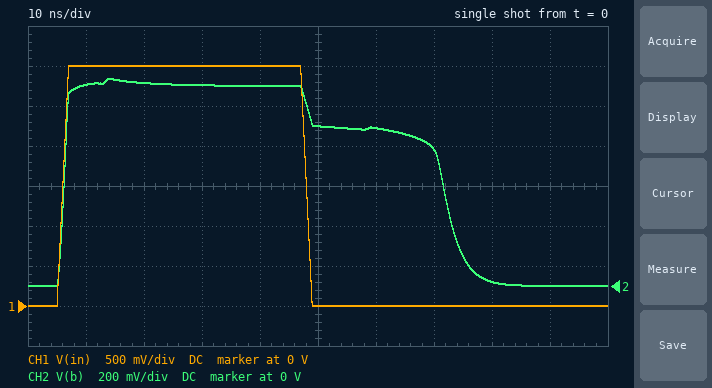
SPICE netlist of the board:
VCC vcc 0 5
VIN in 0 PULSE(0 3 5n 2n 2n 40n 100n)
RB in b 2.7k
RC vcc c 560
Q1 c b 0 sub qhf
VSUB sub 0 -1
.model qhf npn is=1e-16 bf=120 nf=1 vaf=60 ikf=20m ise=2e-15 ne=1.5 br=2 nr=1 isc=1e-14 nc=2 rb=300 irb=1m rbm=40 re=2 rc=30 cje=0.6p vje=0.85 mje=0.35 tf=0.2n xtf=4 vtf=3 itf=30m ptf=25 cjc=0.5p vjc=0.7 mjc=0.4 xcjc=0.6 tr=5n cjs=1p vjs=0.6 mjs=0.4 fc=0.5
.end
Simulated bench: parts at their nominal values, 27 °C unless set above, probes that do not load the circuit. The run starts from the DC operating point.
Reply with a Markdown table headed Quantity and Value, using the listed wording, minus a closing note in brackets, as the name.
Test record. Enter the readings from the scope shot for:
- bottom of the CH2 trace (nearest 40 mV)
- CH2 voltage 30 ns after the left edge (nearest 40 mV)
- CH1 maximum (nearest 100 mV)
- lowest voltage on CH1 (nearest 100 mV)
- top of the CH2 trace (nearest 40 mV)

| Quantity | Value |
|---|---|
| bottom of the CH2 trace | 0 V |
| CH2 voltage 30 ns after the left edge | 1.00 V |
| CH1 maximum | 3.0 V |
| lowest voltage on CH1 | 0 V |
| top of the CH2 trace | 1.04 V |
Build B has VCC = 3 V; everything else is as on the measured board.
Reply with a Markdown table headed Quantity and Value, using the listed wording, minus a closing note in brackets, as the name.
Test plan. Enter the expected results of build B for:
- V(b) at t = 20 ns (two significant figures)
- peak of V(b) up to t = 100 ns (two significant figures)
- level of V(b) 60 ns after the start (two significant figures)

| Quantity | Value |
|---|---|
| V(b) at t = 20 ns | 990 mV |
| peak of V(b) up to t = 100 ns | 1.0 V |
| level of V(b) 60 ns after the start | 760 mV |
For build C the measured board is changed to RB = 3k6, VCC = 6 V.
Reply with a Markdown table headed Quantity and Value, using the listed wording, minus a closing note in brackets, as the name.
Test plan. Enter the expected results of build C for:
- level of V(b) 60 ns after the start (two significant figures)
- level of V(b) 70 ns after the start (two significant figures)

| Quantity | Value |
|---|---|
| level of V(b) 60 ns after the start | 810 mV |
| level of V(b) 70 ns after the start | 760 mV |
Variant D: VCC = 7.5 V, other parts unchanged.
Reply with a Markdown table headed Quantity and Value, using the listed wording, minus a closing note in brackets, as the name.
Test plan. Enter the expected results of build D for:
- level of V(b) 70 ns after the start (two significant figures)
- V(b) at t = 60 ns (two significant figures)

| Quantity | Value |
|---|---|
| level of V(b) 70 ns after the start | 750 mV |
| V(b) at t = 60 ns | 810 mV |
